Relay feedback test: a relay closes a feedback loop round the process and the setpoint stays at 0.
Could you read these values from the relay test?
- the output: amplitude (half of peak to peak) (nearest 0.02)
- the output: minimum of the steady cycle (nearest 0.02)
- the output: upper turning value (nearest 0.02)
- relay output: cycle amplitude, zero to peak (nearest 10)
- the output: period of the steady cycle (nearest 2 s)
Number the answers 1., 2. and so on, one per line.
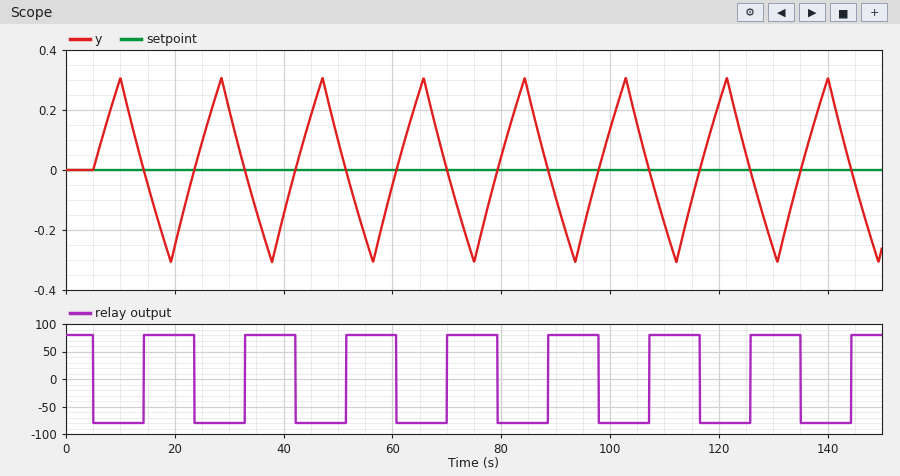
1. 0.30
2. -0.30
3. 0.30
4. 80
5. 18 s
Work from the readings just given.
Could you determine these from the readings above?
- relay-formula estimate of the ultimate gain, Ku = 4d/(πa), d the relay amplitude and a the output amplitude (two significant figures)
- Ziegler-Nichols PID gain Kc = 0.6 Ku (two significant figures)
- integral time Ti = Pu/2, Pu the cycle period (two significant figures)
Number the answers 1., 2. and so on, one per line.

1. 340
2. 200
3. 9.0 s
